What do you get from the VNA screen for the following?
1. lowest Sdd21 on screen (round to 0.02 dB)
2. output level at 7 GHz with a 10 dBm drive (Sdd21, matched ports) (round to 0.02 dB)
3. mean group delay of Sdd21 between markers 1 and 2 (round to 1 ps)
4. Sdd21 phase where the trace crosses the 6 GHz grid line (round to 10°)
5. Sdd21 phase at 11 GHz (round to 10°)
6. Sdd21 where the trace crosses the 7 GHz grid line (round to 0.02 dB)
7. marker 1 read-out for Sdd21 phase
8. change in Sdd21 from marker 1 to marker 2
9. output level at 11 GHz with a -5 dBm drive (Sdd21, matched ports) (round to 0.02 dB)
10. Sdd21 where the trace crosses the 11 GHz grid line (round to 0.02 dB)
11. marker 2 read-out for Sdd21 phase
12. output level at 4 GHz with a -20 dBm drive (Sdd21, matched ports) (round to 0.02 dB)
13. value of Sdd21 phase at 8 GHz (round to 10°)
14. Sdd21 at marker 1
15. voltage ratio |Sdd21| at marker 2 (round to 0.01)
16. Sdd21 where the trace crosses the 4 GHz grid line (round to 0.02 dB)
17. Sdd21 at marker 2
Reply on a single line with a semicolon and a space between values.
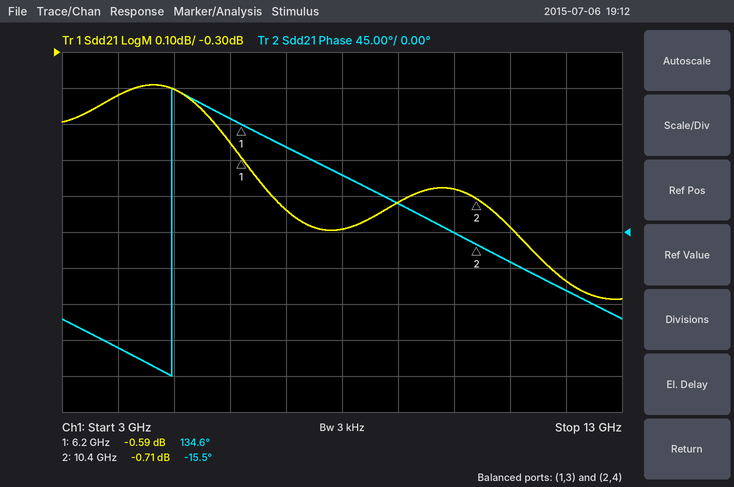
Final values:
-0.98 dB; 9.26 dBm; 99 ps; 140°; -40°; -0.74 dB; 134.6°; -0.12 dB; -5.78 dBm; -0.78 dB; -15.5°; -20.42 dBm; 70°; -0.59 dB; 0.92; -0.42 dB; -0.71 dB
